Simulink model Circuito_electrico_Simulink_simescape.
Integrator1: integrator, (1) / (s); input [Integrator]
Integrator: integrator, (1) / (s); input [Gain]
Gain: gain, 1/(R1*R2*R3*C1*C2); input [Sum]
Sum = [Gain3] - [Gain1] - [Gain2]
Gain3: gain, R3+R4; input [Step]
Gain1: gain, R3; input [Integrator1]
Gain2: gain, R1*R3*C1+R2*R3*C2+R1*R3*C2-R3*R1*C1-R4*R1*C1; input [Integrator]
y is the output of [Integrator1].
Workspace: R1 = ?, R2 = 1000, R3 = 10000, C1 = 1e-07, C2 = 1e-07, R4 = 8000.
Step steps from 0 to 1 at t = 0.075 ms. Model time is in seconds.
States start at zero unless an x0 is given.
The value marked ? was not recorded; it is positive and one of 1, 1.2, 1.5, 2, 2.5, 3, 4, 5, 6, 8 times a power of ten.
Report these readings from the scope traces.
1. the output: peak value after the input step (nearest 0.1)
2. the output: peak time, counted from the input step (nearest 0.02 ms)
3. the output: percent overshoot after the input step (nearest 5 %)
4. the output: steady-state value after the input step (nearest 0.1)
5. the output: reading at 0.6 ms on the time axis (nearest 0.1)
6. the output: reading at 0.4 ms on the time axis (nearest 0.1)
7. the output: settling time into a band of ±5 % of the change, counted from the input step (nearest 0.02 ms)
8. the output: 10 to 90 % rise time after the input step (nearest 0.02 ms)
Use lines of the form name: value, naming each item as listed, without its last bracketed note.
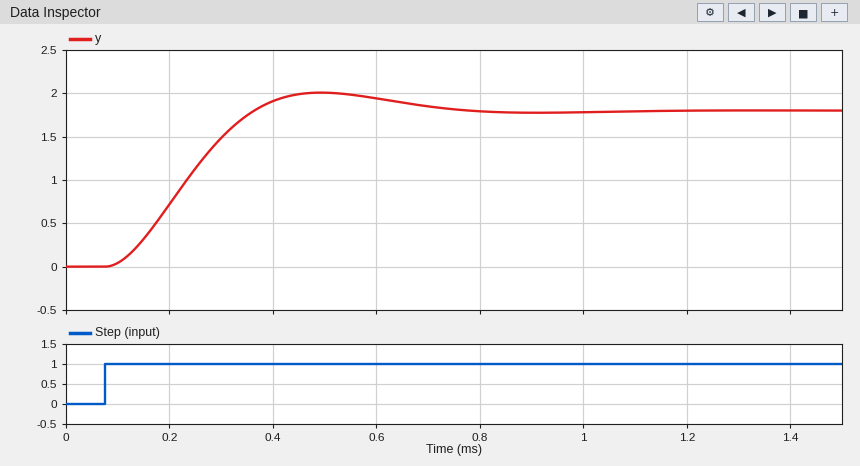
the output: peak value after the input step: 2.0
the output: peak time, counted from the input step: 0.42 ms
the output: percent overshoot after the input step: 10 %
the output: steady-state value after the input step: 1.8
the output: reading at 0.6 ms on the time axis: 1.9
the output: reading at 0.4 ms on the time axis: 1.9
the output: settling time into a band of ±5 % of the change, counted from the input step: 0.58 ms
the output: 10 to 90 % rise time after the input step: 0.20 ms
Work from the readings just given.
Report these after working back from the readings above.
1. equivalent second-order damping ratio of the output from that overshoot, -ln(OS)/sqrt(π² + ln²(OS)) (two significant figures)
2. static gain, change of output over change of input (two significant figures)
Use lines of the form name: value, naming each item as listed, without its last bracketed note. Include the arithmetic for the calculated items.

equivalent second-order damping ratio of the output from that overshoot, -ln(OS)/sqrt(π² + ln²(OS)): ln(0.1) = -2.303; 2.303 / sqrt(9.870 + 5.302) = 0.59
static gain, change of output over change of input: (1.8 - 0) / (1 - 0) = 1.8
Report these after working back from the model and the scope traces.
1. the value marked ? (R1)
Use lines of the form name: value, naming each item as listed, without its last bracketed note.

the value marked ?: 1200
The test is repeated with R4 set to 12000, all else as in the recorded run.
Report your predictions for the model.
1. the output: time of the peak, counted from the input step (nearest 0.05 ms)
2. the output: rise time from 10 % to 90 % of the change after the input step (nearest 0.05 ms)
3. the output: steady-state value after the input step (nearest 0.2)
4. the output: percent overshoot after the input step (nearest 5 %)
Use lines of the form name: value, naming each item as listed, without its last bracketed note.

the output: time of the peak, counted from the input step: 0.35 ms
the output: rise time from 10 % to 90 % of the change after the input step: 0.15 ms
the output: steady-state value after the input step: 2.2
the output: percent overshoot after the input step: 30 %
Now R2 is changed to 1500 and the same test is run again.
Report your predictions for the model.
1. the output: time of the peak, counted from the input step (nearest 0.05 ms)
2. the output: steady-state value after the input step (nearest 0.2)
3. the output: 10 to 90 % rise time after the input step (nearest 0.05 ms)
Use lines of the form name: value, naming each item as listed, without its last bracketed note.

the output: time of the peak, counted from the input step: 0.55 ms
the output: steady-state value after the input step: 1.8
the output: 10 to 90 % rise time after the input step: 0.25 ms
